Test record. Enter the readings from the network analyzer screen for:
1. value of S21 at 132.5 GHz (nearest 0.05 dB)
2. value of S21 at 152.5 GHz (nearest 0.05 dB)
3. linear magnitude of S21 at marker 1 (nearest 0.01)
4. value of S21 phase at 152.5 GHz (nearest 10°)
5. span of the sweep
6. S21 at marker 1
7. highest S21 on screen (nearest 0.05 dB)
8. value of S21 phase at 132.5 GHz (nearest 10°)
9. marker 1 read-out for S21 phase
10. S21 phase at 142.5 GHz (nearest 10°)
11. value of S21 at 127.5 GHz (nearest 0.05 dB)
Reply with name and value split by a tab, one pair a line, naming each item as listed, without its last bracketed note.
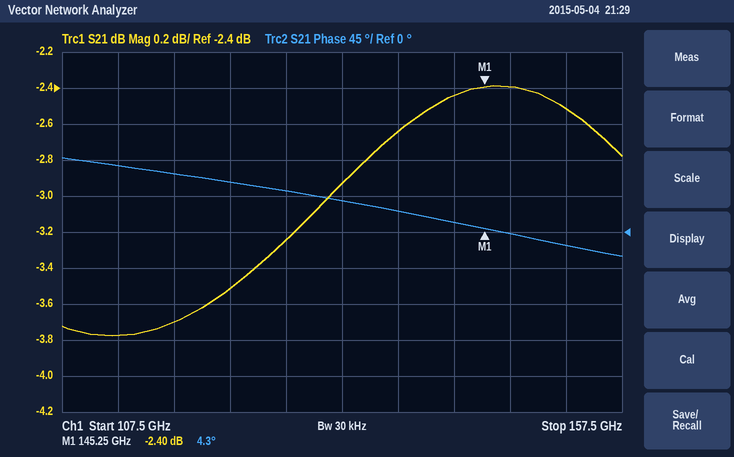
value of S21 at 132.5 GHz	-2.95 dB
value of S21 at 152.5 GHz	-2.50 dB
linear magnitude of S21 at marker 1	0.76
value of S21 phase at 152.5 GHz	-20°
span of the sweep	50 GHz
S21 at marker 1	-2.40 dB
highest S21 on screen	-2.40 dB
value of S21 phase at 132.5 GHz	40°
marker 1 read-out for S21 phase	4.3°
S21 phase at 142.5 GHz	10°
value of S21 at 127.5 GHz	-3.25 dB
